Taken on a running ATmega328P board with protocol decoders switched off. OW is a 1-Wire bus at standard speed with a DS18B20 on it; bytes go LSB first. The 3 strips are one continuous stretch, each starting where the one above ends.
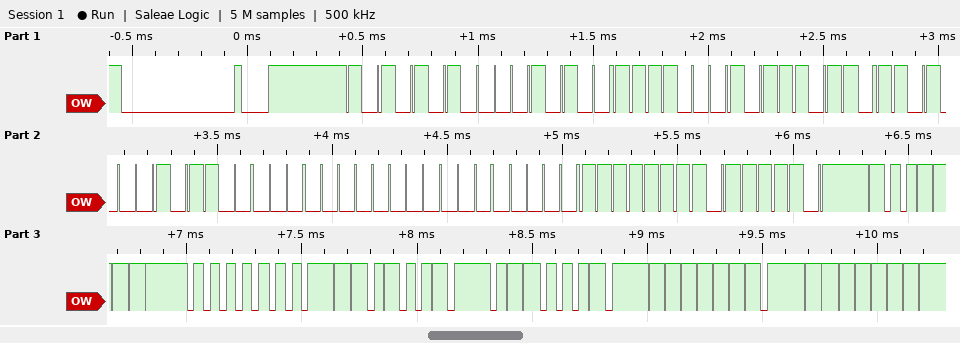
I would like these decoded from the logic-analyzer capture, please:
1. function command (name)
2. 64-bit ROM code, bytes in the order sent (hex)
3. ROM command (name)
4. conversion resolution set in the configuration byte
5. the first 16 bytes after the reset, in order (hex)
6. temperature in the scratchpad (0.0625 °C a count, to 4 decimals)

Read Scratchpad
28 8F 6E 8B 06 00 00 FF
Match ROM
12 bits
55 28 8F 6E 8B 06 00 00 FF BE F9 00 4B 46 7F FF
15.5625 °C
